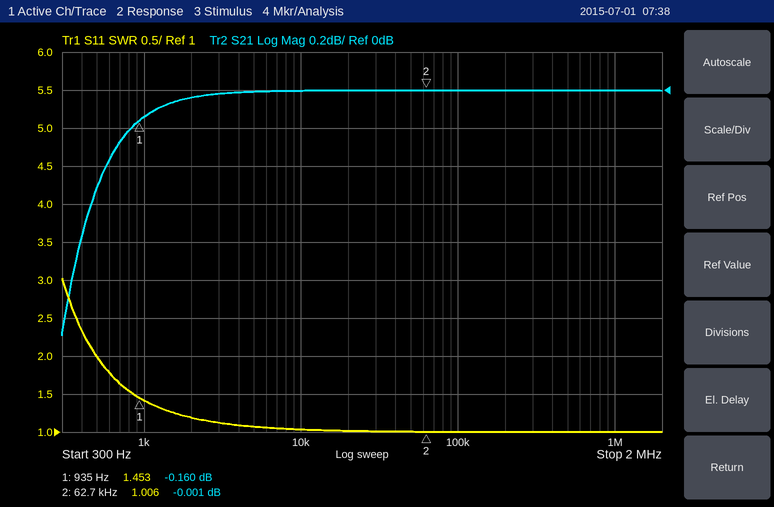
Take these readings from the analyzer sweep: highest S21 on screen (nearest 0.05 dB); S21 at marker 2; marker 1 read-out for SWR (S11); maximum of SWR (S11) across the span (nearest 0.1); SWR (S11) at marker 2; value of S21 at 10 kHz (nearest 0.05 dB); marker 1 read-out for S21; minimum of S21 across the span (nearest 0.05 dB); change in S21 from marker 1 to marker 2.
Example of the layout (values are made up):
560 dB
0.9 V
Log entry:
0.00 dB
-0.001 dB
1.453
3.0
1.006
0.00 dB
-0.160 dB
-1.30 dB
0.159 dB
